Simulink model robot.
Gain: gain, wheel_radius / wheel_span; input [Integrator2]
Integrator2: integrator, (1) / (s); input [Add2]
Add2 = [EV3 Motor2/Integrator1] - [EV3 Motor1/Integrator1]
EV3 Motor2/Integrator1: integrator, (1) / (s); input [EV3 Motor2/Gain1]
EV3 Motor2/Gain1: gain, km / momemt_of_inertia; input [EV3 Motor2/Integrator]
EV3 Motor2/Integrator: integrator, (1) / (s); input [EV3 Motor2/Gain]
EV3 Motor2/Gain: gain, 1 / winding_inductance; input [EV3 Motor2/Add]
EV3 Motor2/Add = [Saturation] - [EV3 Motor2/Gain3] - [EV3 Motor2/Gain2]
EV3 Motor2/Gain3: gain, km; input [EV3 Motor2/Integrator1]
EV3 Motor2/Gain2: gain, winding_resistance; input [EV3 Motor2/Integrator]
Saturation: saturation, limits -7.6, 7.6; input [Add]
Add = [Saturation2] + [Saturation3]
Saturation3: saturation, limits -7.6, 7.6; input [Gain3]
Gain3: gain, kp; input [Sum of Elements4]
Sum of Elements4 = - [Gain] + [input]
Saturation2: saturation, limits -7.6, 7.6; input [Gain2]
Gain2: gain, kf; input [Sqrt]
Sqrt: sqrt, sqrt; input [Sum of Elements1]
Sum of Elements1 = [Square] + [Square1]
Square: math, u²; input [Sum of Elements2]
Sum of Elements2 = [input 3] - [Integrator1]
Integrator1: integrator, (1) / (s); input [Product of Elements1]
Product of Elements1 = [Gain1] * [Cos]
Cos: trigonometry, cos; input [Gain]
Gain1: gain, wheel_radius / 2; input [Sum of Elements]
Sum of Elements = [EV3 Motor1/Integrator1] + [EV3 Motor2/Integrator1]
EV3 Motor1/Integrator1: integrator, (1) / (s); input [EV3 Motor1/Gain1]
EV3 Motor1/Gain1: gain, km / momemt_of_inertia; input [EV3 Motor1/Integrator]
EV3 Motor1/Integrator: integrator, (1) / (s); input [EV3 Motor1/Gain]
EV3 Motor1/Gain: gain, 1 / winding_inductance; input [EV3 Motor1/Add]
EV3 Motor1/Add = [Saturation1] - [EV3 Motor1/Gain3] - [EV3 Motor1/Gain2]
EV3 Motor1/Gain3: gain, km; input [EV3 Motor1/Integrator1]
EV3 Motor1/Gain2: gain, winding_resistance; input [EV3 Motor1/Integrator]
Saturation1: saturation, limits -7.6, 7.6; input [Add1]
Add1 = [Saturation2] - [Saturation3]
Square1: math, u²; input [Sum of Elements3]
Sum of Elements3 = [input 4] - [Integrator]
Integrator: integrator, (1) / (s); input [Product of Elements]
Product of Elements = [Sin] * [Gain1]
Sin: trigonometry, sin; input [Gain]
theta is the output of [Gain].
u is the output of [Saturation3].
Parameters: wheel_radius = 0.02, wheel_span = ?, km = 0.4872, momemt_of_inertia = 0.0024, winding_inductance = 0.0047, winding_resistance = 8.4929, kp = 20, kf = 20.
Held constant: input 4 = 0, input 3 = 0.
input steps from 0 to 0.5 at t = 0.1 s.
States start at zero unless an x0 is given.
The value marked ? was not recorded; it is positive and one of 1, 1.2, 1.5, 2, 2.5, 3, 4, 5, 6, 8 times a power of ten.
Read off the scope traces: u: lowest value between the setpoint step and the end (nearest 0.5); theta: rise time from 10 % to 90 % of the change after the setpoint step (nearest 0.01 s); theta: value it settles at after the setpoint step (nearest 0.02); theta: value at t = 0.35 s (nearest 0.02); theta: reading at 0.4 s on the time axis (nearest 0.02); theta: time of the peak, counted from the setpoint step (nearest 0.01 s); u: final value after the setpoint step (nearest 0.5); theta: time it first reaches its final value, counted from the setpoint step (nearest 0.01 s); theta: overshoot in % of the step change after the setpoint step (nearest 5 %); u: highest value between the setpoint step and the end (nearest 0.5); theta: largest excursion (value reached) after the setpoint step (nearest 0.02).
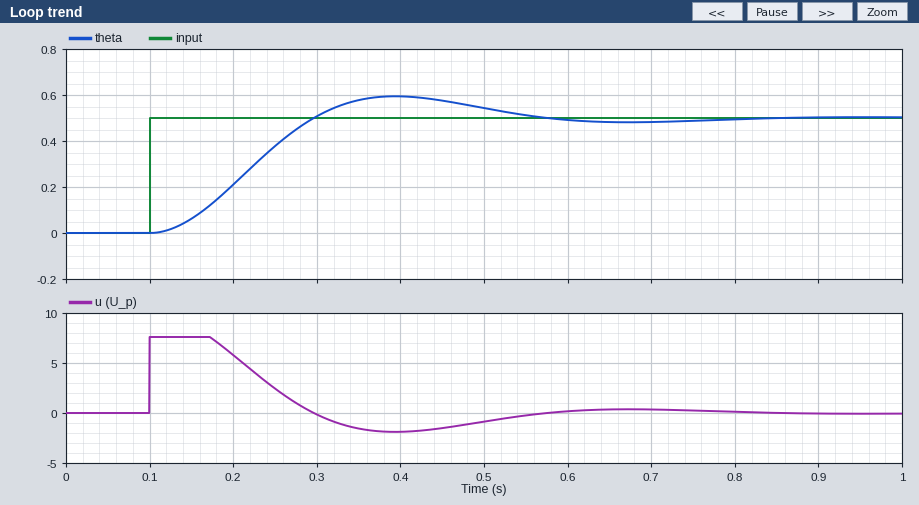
-2.0
0.13 s
0.50
0.58
0.60
0.29 s
0.0
0.20 s
20 %
7.5
0.60
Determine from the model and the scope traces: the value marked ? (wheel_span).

0.12
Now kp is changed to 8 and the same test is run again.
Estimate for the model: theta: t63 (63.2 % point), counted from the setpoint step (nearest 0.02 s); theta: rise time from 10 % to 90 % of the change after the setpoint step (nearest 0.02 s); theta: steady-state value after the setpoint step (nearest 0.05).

0.22 s
0.28 s
0.50
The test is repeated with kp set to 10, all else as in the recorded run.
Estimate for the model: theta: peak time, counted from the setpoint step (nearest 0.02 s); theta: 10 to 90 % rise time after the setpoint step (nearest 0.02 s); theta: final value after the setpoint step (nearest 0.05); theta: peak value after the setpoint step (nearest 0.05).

0.46 s
0.22 s
0.50
0.55
